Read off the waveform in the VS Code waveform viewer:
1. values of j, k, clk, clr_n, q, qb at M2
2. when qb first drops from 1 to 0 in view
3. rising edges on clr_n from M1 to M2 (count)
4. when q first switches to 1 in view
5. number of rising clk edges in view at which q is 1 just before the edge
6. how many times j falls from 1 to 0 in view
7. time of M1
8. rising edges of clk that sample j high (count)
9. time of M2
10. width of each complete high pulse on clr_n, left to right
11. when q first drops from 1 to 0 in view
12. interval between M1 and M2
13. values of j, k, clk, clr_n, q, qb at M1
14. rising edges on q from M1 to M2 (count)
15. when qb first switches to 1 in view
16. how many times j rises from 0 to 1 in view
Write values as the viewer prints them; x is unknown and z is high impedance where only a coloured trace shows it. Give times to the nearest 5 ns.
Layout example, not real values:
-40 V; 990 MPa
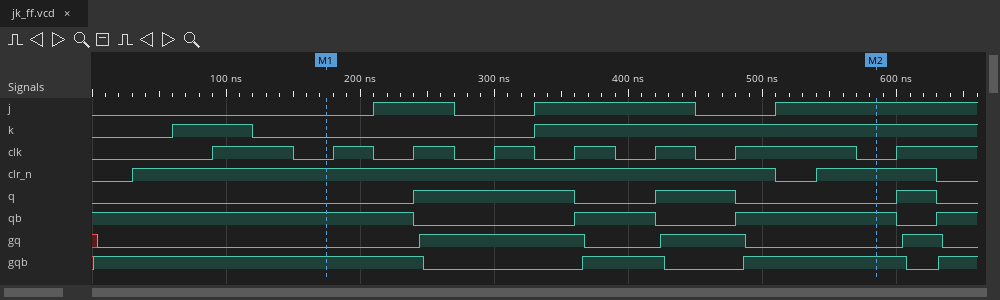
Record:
j=1, k=1, clk=0, clr_n=1, q=0, qb=1; 240 ns; 1; 240 ns; 3; 2; 175 ns; 4; 585 ns; 480 ns, 90 ns; 360 ns; 410 ns; j=0, k=0, clk=0, clr_n=1, q=0, qb=1; 2; 360 ns; 3
